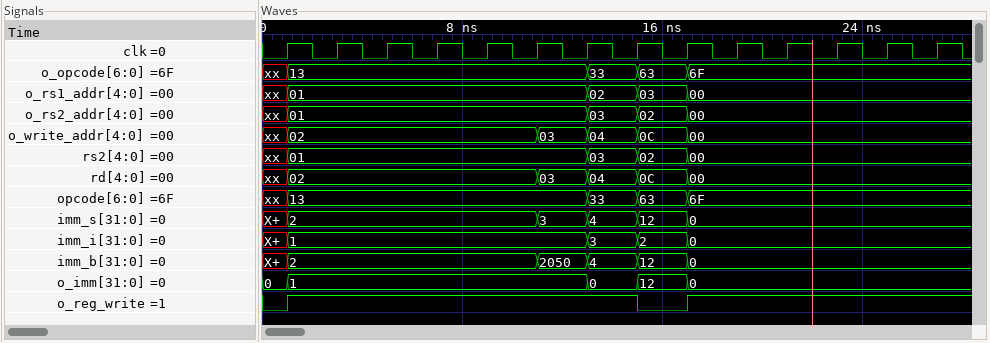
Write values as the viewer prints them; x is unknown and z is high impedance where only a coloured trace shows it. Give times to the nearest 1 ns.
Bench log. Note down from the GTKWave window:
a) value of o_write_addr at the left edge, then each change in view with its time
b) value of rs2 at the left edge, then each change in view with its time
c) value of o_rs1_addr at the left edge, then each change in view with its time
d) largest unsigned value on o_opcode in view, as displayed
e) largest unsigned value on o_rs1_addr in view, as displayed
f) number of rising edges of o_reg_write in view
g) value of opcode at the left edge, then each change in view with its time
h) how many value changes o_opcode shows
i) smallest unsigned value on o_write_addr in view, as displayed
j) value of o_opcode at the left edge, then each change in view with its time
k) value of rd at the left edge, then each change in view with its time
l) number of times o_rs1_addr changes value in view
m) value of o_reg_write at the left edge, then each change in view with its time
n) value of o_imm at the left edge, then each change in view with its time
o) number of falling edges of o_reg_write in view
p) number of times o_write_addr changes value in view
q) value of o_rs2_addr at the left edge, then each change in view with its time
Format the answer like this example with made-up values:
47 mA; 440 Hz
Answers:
xx, 02 at 1 ns, 03 at 11 ns, 04 at 13 ns, 0C at 15 ns, 00 at 17 ns; xx, 01 at 1 ns, 03 at 13 ns, 02 at 15 ns, 00 at 17 ns; xx, 01 at 1 ns, 02 at 13 ns, 03 at 15 ns, 00 at 17 ns; 6F; 03; 2; xx, 13 at 1 ns, 33 at 13 ns, 63 at 15 ns, 6F at 17 ns; 4; 00; xx, 13 at 1 ns, 33 at 13 ns, 63 at 15 ns, 6F at 17 ns; xx, 02 at 1 ns, 03 at 11 ns, 04 at 13 ns, 0C at 15 ns, 00 at 17 ns; 4; 0, 1 at 1 ns, 0 at 15 ns, 1 at 17 ns; 0, 1 at 1 ns, 0 at 13 ns, 12 at 15 ns, 0 at 17 ns; 1; 5; xx, 01 at 1 ns, 03 at 13 ns, 02 at 15 ns, 00 at 17 ns
